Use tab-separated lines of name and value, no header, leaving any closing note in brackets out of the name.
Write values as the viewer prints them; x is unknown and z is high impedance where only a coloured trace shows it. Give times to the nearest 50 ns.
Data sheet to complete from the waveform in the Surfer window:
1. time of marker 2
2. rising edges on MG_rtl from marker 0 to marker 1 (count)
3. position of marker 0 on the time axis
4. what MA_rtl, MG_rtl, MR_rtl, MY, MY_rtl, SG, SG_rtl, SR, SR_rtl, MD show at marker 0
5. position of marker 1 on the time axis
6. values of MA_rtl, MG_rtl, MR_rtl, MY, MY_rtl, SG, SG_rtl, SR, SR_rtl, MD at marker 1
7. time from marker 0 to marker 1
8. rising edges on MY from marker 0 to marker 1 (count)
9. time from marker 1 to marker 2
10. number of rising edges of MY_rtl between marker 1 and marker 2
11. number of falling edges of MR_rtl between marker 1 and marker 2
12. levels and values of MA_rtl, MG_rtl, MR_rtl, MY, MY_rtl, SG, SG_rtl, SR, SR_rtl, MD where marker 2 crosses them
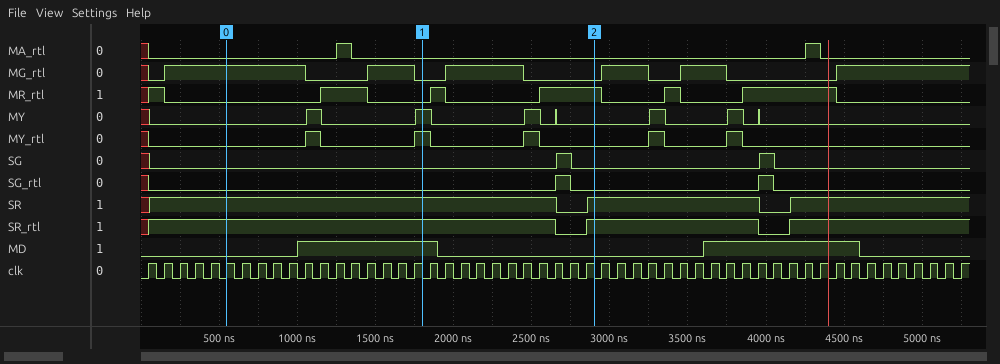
time of marker 2	2900 ns
rising edges on MG_rtl from marker 0 to marker 1	1
position of marker 0 on the time axis	550 ns
what MA_rtl, MG_rtl, MR_rtl, MY, MY_rtl, SG, SG_rtl, SR, SR_rtl, MD show at marker 0	MA_rtl=0, MG_rtl=1, MR_rtl=0, MY=0, MY_rtl=0, SG=0, SG_rtl=0, SR=1, SR_rtl=1, MD=0
position of marker 1 on the time axis	1800 ns
values of MA_rtl, MG_rtl, MR_rtl, MY, MY_rtl, SG, SG_rtl, SR, SR_rtl, MD at marker 1	MA_rtl=0, MG_rtl=0, MR_rtl=0, MY=1, MY_rtl=1, SG=0, SG_rtl=0, SR=1, SR_rtl=1, MD=1
time from marker 0 to marker 1	1250 ns
rising edges on MY from marker 0 to marker 1	2
time from marker 1 to marker 2	1100 ns
number of rising edges of MY_rtl between marker 1 and marker 2	1
number of falling edges of MR_rtl between marker 1 and marker 2	1
levels and values of MA_rtl, MG_rtl, MR_rtl, MY, MY_rtl, SG, SG_rtl, SR, SR_rtl, MD where marker 2 crosses them	MA_rtl=0, MG_rtl=0, MR_rtl=1, MY=0, MY_rtl=0, SG=0, SG_rtl=0, SR=1, SR_rtl=1, MD=0
